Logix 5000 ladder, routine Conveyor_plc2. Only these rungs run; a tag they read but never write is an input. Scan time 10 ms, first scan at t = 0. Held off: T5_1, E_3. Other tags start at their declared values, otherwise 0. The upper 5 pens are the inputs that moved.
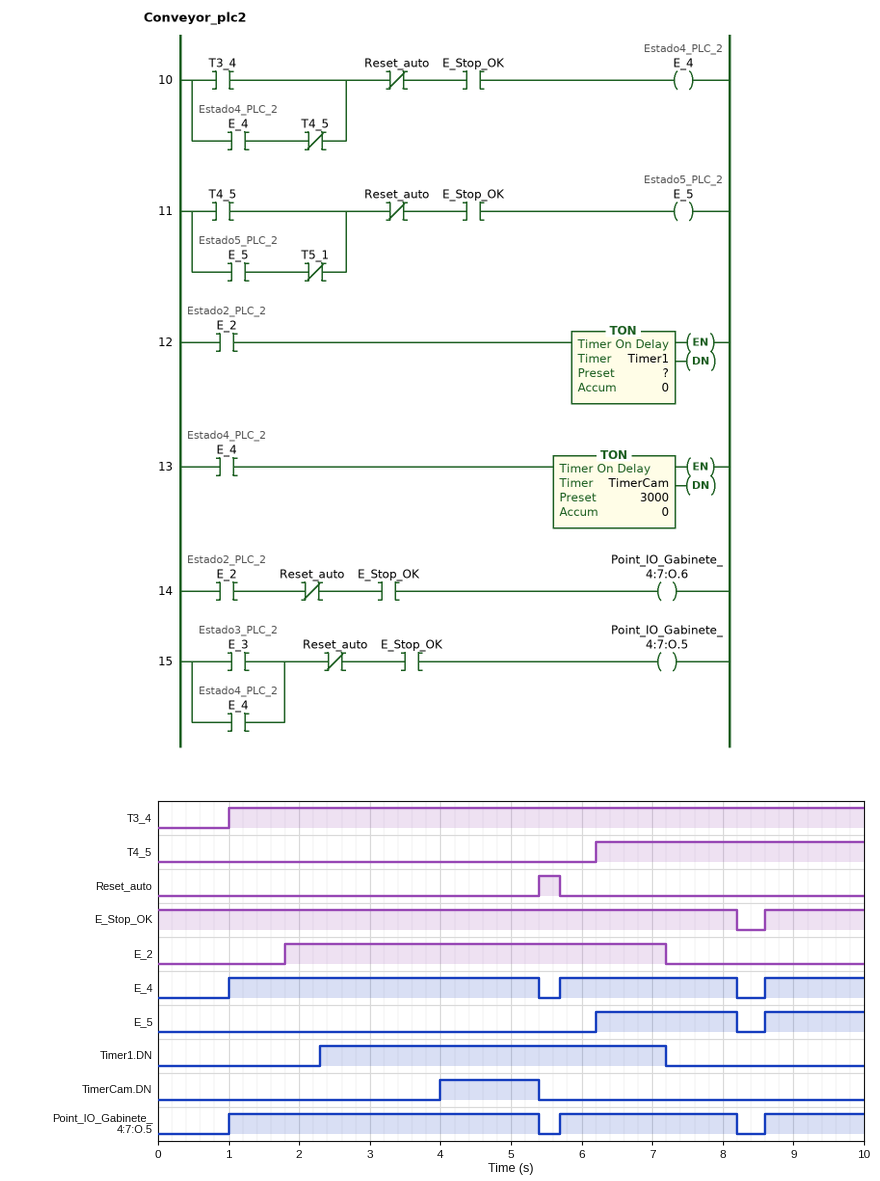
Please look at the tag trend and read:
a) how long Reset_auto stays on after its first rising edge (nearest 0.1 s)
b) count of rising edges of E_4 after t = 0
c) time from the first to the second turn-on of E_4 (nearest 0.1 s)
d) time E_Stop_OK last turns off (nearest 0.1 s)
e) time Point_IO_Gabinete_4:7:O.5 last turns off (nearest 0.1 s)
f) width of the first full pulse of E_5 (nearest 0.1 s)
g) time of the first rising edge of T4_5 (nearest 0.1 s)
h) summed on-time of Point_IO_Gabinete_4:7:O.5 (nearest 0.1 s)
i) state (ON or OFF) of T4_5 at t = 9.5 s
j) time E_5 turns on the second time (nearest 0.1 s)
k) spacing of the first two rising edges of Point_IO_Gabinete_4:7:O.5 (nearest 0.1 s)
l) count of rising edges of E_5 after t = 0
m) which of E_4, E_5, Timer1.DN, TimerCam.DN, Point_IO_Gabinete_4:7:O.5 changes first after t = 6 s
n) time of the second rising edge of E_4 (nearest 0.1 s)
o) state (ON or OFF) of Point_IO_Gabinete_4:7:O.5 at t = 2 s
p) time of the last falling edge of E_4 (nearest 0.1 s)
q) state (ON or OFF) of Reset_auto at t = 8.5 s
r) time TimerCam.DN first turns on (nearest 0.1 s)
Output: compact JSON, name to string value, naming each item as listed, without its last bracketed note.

{"how long Reset_auto stays on after its first rising edge": "0.3 s", "count of rising edges of E_4 after t = 0": "3", "time from the first to the second turn-on of E_4": "4.7 s", "time E_Stop_OK last turns off": "8.2 s", "time Point_IO_Gabinete_4:7:O.5 last turns off": "8.2 s", "width of the first full pulse of E_5": "2.0 s", "time of the first rising edge of T4_5": "6.2 s", "summed on-time of Point_IO_Gabinete_4:7:O.5": "8.3 s", "state (ON or OFF) of T4_5 at t = 9.5 s": "ON", "time E_5 turns on the second time": "8.6 s", "spacing of the first two rising edges of Point_IO_Gabinete_4:7:O.5": "4.7 s", "count of rising edges of E_5 after t = 0": "2", "which of E_4, E_5, Timer1.DN, TimerCam.DN, Point_IO_Gabinete_4:7:O.5 changes first after t = 6 s": "E_5", "time of the second rising edge of E_4": "5.7 s", "state (ON or OFF) of Point_IO_Gabinete_4:7:O.5 at t = 2 s": "ON", "time of the last falling edge of E_4": "8.2 s", "state (ON or OFF) of Reset_auto at t = 8.5 s": "OFF", "time TimerCam.DN first turns on": "4.0 s"}
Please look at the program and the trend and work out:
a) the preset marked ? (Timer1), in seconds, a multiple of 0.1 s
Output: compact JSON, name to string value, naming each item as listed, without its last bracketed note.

{"the preset marked ? (Timer1), in seconds, a multiple of 0.1 s": "0.5 s"}
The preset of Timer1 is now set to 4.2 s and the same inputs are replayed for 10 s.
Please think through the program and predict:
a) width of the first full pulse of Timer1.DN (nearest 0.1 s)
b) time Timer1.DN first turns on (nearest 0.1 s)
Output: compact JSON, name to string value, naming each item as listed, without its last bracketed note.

{"width of the first full pulse of Timer1.DN": "1.2 s", "time Timer1.DN first turns on": "6.0 s"}
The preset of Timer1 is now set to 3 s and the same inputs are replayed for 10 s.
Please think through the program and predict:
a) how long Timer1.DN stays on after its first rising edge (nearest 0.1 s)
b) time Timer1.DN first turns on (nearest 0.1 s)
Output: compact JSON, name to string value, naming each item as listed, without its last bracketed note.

{"how long Timer1.DN stays on after its first rising edge": "2.4 s", "time Timer1.DN first turns on": "4.8 s"}
